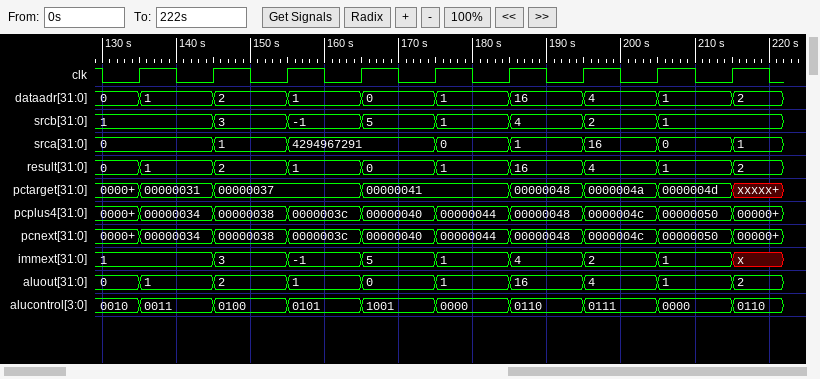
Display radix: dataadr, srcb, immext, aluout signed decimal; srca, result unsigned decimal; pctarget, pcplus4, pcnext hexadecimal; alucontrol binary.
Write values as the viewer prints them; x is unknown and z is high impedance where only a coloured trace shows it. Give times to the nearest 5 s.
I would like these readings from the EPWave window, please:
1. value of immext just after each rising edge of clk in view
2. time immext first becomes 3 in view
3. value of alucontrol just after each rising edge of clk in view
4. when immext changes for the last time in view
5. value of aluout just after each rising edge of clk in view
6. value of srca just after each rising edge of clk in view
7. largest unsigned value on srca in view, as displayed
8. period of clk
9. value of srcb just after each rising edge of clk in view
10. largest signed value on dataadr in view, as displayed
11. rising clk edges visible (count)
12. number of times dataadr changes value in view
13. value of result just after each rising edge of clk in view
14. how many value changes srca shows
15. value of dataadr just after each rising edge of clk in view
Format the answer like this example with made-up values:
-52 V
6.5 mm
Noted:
1, 3, -1, 5, 1, 4, 2, 1, x
145 s
0011, 0100, 0101, 1001, 0000, 0110, 0111, 0000, 0110
215 s
1, 2, 1, 0, 1, 16, 4, 1, 2
0, 1, 4294967291, 4294967291, 0, 1, 16, 0, 1
4294967291
10 s
1, 3, -1, 5, 1, 4, 2, 1, 1
16
9
9
1, 2, 1, 0, 1, 16, 4, 1, 2
7
1, 2, 1, 0, 1, 16, 4, 1, 2
